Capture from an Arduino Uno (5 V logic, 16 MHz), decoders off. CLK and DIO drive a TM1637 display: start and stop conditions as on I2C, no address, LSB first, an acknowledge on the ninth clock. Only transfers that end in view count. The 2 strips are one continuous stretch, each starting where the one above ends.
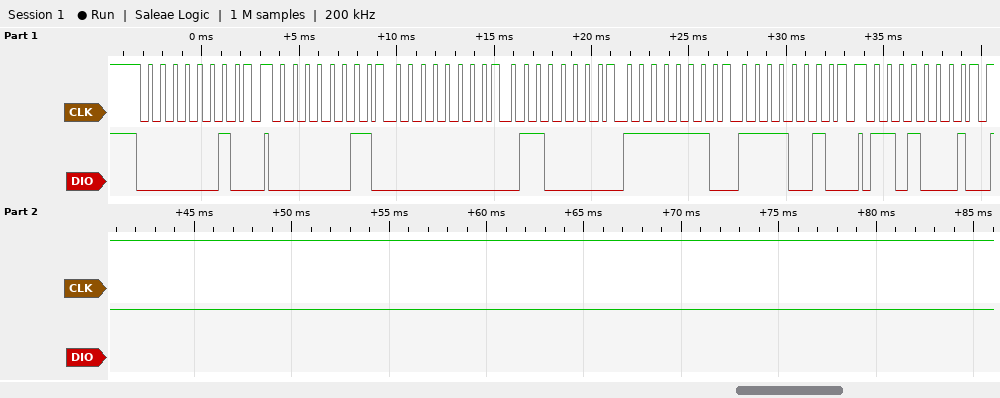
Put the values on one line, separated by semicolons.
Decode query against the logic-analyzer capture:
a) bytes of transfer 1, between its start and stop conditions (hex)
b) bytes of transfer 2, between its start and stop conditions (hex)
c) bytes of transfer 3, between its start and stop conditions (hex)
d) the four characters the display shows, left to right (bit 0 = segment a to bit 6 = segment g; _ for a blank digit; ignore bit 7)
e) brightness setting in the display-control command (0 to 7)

40; C0 00 06 7F 4F; 8B; _183; 3
